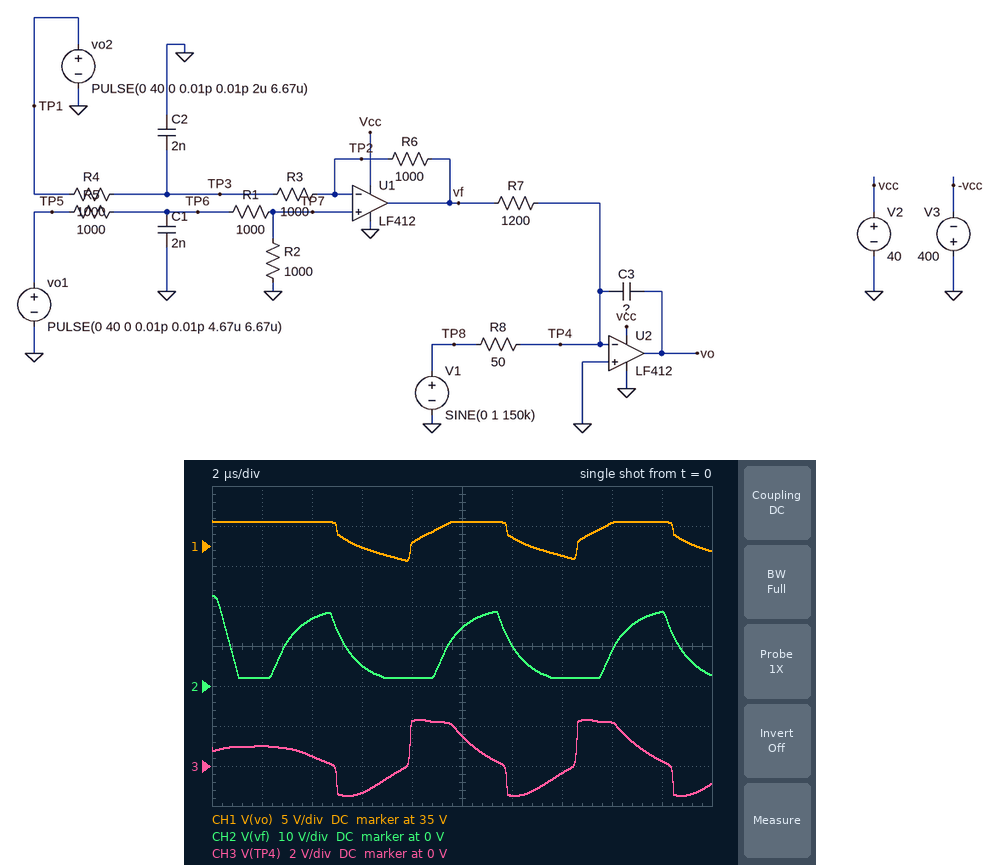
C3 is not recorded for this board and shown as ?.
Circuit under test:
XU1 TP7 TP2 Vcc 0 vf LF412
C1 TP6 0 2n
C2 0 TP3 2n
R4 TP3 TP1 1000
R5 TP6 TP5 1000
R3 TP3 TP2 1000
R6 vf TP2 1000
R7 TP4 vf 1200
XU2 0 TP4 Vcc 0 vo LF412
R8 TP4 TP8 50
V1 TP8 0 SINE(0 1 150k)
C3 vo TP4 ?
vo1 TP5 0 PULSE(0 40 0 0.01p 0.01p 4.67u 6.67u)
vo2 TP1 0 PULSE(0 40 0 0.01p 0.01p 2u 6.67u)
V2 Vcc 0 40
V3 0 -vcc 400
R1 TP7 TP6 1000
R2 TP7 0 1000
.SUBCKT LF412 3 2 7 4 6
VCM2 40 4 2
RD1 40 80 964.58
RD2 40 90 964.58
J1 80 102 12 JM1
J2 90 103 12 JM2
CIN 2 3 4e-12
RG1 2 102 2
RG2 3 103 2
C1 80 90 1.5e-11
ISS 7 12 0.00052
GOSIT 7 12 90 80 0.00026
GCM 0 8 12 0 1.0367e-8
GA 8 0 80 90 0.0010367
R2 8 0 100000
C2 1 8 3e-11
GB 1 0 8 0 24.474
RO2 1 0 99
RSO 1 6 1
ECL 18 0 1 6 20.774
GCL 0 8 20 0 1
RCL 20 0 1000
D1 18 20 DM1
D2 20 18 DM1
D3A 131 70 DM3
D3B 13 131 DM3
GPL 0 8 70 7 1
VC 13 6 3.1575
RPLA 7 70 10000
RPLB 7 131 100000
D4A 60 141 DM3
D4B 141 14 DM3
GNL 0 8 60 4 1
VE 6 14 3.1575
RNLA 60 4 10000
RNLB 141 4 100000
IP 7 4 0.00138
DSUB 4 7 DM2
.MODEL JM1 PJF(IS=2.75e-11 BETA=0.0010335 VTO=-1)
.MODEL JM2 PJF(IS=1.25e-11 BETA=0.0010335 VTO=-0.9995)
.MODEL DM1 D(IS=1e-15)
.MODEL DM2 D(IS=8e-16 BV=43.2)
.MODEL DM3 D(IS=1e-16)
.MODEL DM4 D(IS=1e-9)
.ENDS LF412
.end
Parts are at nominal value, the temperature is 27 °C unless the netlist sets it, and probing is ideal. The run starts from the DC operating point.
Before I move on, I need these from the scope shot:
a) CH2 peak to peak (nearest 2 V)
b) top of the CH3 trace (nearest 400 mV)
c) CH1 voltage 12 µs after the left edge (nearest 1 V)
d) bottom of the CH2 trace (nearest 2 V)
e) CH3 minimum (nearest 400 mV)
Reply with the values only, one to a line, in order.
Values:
20 V
2.4 V
36 V
2 V
-1.6 V
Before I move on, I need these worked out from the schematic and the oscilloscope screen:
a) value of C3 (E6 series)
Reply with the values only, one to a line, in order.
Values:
15 nF
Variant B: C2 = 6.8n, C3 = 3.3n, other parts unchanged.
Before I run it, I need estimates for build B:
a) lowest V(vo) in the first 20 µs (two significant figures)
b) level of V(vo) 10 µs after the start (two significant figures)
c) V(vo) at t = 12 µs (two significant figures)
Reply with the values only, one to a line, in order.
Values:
14 V
35 V
29 V
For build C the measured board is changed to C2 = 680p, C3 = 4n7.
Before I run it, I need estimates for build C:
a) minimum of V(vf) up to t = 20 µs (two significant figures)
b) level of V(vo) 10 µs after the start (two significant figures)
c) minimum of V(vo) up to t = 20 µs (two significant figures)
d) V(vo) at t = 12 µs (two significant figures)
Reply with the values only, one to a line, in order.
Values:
2.0 V
36 V
22 V
33 V
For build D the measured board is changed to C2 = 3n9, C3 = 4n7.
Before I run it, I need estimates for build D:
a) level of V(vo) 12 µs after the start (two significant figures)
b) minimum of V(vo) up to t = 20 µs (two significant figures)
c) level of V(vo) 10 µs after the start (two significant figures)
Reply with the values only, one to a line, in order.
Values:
32 V
21 V
36 V
